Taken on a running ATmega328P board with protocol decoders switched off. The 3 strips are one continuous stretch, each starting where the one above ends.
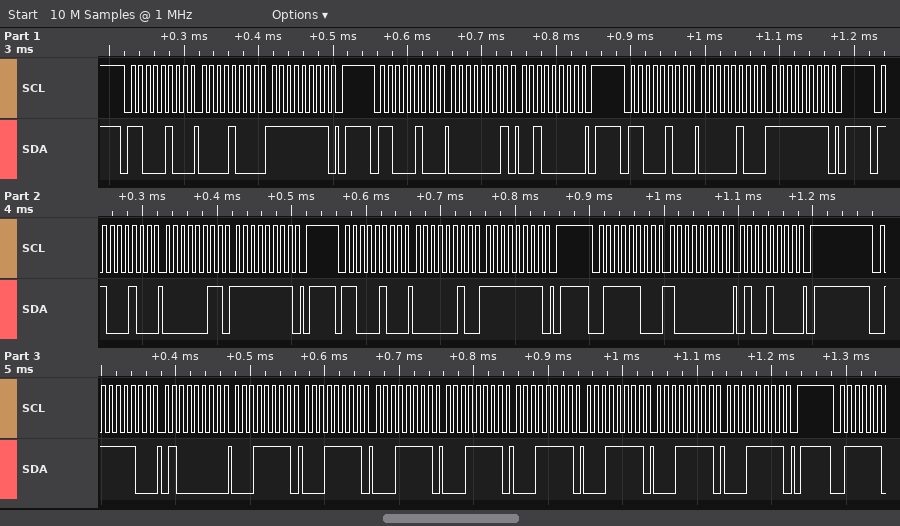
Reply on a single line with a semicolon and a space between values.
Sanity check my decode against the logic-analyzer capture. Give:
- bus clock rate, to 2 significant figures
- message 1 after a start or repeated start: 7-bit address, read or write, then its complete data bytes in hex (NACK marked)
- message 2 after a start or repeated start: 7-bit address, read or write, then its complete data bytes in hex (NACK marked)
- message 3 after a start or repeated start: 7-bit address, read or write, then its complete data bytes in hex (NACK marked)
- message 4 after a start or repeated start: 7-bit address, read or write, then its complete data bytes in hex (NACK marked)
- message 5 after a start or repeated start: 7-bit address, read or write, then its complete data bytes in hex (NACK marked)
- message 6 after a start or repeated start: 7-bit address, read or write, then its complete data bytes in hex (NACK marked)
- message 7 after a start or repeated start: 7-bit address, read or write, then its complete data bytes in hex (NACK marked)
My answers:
100 kHz; 0x62 write: 08 FF; 0x62 write: 01 20; 0x62 write: 04 FF; 0x62 write: 03 FF; 0x62 write: 02 FF; 0x3E write: 80 48; 0x3E write: 40 1F 1F 1F 1F 1F 1F 1F 1F
